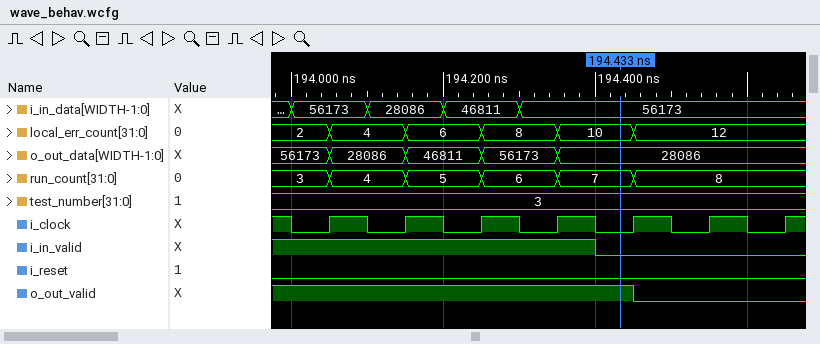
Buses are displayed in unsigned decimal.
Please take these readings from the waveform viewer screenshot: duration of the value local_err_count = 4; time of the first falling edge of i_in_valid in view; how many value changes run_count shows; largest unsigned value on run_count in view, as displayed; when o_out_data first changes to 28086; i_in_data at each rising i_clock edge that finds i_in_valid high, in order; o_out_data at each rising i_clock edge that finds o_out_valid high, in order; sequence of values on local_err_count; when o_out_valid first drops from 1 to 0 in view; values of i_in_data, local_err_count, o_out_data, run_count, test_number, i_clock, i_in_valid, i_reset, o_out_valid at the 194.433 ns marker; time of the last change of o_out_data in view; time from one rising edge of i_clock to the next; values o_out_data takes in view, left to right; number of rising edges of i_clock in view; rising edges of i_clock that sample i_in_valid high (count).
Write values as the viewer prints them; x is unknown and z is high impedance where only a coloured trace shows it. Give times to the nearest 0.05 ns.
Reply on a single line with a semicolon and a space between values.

0.1 ns; 194.4 ns; 5; 8; 194.05 ns; 56173, 28086, 46811, 56173; 56173, 28086, 46811, 56173, 28086; 2, 4, 6, 8, 10, 12; 194.45 ns; i_in_data=56173, local_err_count=10, o_out_data=28086, run_count=7, test_number=3, i_clock=0, i_in_valid=0, i_reset=0, o_out_valid=1; 194.35 ns; 0.1 ns; 56173, 28086, 46811, 56173, 28086; 7; 4
